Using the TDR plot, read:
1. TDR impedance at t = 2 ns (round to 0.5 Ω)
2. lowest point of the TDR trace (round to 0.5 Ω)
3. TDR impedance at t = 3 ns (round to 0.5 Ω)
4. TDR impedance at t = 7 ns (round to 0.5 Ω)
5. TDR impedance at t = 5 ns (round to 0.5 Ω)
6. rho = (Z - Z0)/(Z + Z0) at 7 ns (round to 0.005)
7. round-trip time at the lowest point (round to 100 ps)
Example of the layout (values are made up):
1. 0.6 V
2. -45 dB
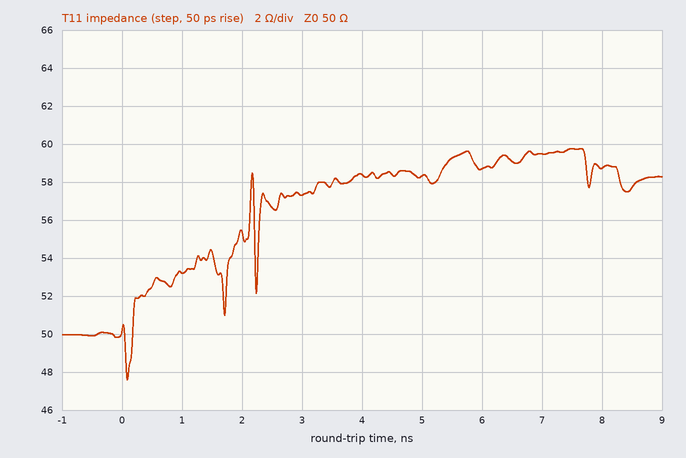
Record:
1. 55.5 Ω
2. 47.5 Ω
3. 57.5 Ω
4. 59.5 Ω
5. 58.5 Ω
6. +0.085
7. 100 ps
